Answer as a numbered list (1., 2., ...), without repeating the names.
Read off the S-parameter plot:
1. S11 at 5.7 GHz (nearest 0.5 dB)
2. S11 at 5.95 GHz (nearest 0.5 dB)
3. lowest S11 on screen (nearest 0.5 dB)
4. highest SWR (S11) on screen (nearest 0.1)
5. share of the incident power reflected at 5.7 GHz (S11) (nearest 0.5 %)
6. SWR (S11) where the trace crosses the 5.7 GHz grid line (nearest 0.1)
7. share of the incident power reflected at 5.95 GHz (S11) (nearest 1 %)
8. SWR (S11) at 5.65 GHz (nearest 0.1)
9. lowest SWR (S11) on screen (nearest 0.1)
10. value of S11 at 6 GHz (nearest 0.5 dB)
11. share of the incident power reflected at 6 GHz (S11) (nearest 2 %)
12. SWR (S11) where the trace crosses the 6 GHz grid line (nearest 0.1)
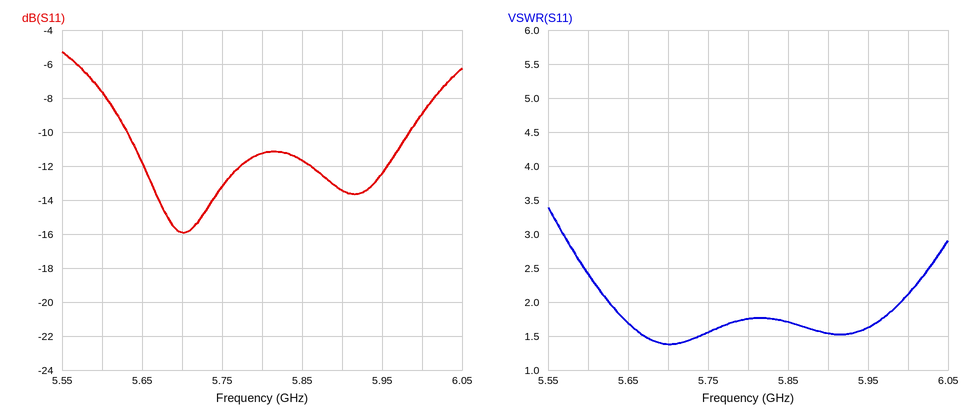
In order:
1. -16.0 dB
2. -12.5 dB
3. -16.0 dB
4. 3.4
5. 2.5 %
6. 1.4
7. 6 %
8. 1.7
9. 1.4
10. -9.0 dB
11. 12 %
12. 2.1
